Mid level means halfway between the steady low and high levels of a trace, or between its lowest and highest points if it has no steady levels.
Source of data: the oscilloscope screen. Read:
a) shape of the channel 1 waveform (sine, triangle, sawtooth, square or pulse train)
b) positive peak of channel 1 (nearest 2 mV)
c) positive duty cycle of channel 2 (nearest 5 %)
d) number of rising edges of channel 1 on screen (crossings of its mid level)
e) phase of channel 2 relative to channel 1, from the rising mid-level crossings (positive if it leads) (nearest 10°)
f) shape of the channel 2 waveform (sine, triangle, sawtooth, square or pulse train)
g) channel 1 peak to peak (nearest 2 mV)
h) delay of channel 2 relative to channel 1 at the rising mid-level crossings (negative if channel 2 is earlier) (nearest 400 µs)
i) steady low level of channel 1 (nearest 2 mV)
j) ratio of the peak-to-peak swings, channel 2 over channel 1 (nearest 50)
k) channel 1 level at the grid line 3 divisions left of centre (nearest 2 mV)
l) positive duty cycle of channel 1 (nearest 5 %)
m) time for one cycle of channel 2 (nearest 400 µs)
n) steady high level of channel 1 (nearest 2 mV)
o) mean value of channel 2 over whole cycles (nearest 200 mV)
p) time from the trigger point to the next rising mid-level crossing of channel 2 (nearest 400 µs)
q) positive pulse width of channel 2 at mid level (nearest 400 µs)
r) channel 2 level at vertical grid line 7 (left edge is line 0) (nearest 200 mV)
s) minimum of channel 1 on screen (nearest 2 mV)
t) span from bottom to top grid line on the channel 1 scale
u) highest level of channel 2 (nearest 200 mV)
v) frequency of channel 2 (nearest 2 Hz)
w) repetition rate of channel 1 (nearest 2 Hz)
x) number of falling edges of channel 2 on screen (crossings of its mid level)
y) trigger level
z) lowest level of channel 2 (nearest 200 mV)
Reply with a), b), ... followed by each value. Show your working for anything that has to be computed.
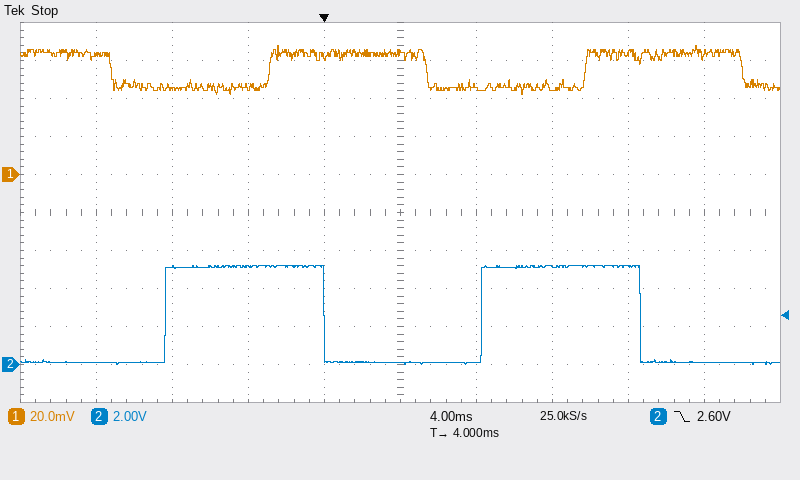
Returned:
a) square
b) 68 mV
c) 8.4 ms / 16.8 ms ≈ 50 %
d) 2
e) −360° × (-5.6 ms) / 16.8 ms ≈ +120°
f) square
g) 68 mV − (42 mV) = 26 mV
h) -5.6 ms
i) 46 mV
j) 5.2 V / 26 mV ≈ 200
k) 46 mV
l) 50 %
m) 16.8 ms
n) 64 mV
o) 0.0 V + 0.5 × (5.2 V − (0.0 V)) ≈ 2.6 V
p) 8.4 ms
q) 8.4 ms
r) 5.2 V
s) 42 mV
t) 200 mV
u) 5.2 V
v) 1 / 16.8 ms ≈ 60 Hz
w) 60 Hz
x) 2
y) 2.60 V
z) 0.0 V
